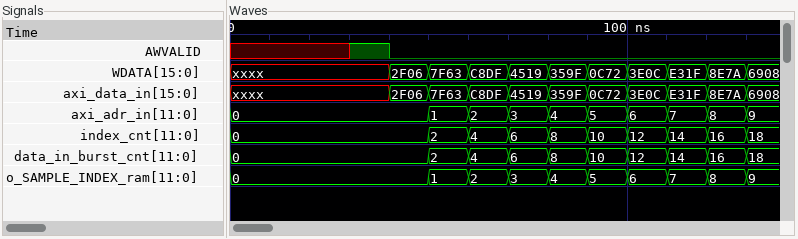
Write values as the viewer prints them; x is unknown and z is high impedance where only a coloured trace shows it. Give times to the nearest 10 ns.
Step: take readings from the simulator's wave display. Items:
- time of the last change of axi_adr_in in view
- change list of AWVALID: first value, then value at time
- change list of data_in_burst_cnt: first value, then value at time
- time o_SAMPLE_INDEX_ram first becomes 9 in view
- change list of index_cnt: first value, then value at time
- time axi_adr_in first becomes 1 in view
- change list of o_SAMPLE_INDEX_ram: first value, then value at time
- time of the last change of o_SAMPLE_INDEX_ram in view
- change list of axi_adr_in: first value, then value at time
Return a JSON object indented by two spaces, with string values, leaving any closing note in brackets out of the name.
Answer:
{
  "time of the last change of axi_adr_in in view": "130 ns",
  "change list of AWVALID: first value, then value at time": "x, 1 at 30 ns, 0 at 40 ns",
  "change list of data_in_burst_cnt: first value, then value at time": "0, 2 at 50 ns, 4 at 60 ns, 6 at 70 ns, 8 at 80 ns, 10 at 90 ns, 12 at 100 ns, 14 at 110 ns, 16 at 120 ns, 18 at 130 ns",
  "time o_SAMPLE_INDEX_ram first becomes 9 in view": "130 ns",
  "change list of index_cnt: first value, then value at time": "0, 2 at 50 ns, 4 at 60 ns, 6 at 70 ns, 8 at 80 ns, 10 at 90 ns, 12 at 100 ns, 14 at 110 ns, 16 at 120 ns, 18 at 130 ns",
  "time axi_adr_in first becomes 1 in view": "50 ns",
  "change list of o_SAMPLE_INDEX_ram: first value, then value at time": "0, 1 at 50 ns, 2 at 60 ns, 3 at 70 ns, 4 at 80 ns, 5 at 90 ns, 6 at 100 ns, 7 at 110 ns, 8 at 120 ns, 9 at 130 ns",
  "time of the last change of o_SAMPLE_INDEX_ram in view": "130 ns",
  "change list of axi_adr_in: first value, then value at time": "0, 1 at 50 ns, 2 at 60 ns, 3 at 70 ns, 4 at 80 ns, 5 at 90 ns, 6 at 100 ns, 7 at 110 ns, 8 at 120 ns, 9 at 130 ns"
}
